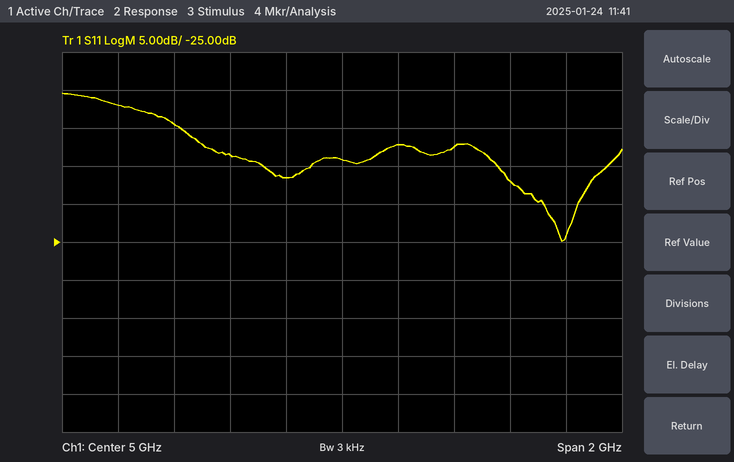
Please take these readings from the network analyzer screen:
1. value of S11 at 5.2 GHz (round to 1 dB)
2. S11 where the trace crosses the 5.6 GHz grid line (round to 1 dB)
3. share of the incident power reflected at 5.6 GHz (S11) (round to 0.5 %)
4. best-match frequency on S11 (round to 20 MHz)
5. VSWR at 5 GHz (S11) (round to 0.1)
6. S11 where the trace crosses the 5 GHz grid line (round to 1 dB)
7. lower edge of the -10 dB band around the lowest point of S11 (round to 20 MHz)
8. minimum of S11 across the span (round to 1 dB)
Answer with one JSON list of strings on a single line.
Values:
["-12 dB", "-17 dB", "2.0 %", "5.78 GHz", "1.5", "-14 dB", "4.42 GHz", "-25 dB"]
